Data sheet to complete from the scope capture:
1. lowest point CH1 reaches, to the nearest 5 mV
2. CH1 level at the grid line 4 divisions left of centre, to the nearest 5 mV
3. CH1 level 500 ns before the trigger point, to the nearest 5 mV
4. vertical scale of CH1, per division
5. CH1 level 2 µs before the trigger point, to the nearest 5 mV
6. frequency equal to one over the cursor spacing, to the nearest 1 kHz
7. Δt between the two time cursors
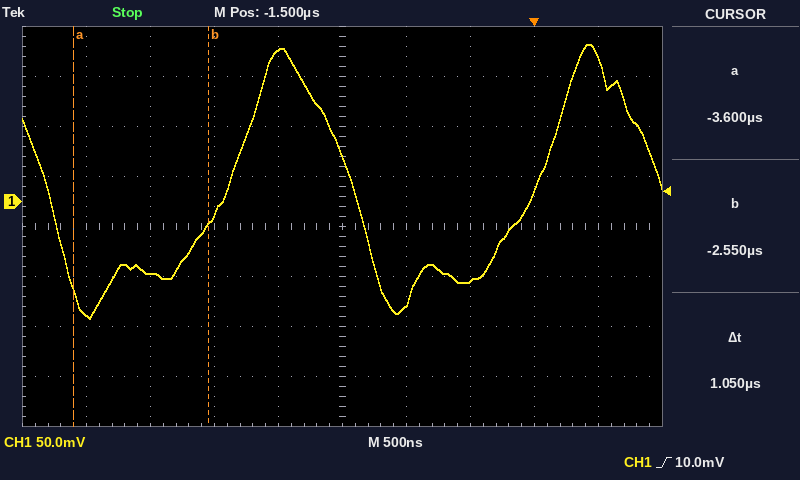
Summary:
-115 mV
-115 mV
-80 mV
50 mV
150 mV
952 kHz
1.05 µs
